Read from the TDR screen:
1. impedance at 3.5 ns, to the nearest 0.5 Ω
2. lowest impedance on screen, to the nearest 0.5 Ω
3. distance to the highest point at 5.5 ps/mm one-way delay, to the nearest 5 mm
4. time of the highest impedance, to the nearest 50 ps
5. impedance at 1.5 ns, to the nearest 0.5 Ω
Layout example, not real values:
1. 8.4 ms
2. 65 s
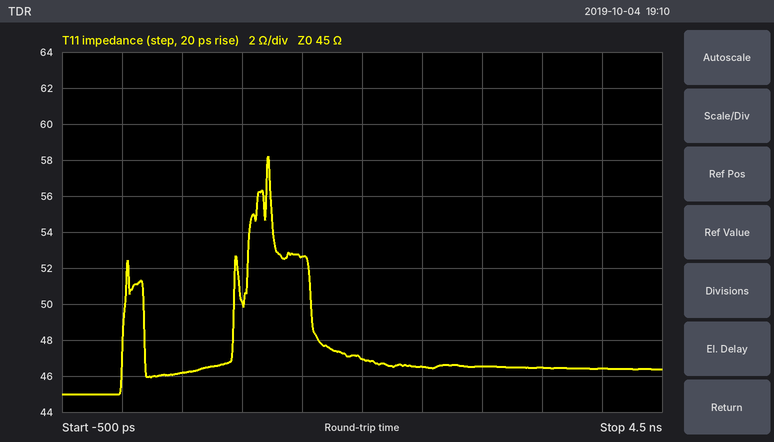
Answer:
1. 46.5 Ω
2. 45.0 Ω
3. 110 mm
4. 1.20 ns
5. 52.5 Ω
